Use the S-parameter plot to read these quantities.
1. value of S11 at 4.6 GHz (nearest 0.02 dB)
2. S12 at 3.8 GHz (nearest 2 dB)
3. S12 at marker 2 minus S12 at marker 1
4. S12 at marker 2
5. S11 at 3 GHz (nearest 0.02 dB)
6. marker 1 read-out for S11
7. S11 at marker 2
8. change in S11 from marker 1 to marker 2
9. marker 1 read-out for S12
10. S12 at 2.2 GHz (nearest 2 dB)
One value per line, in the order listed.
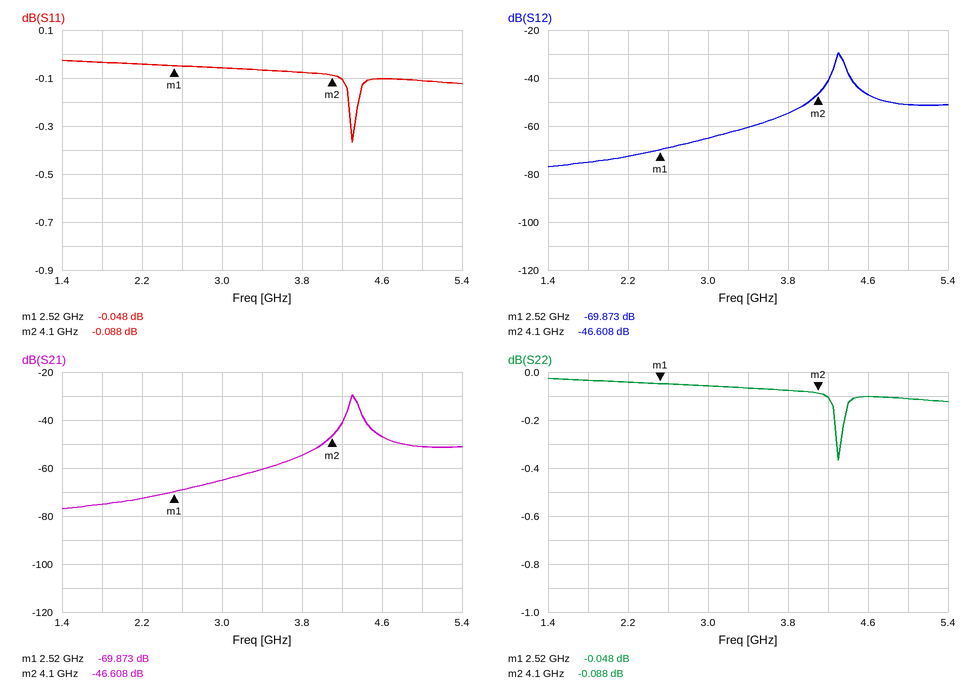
-0.10 dB
-54 dB
23.265 dB
-46.608 dB
-0.06 dB
-0.048 dB
-0.088 dB
-0.040 dB
-69.873 dB
-72 dB
